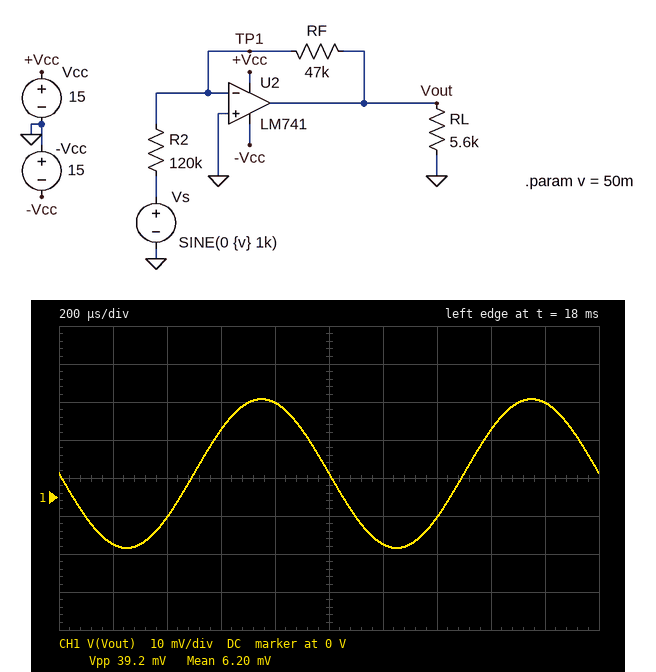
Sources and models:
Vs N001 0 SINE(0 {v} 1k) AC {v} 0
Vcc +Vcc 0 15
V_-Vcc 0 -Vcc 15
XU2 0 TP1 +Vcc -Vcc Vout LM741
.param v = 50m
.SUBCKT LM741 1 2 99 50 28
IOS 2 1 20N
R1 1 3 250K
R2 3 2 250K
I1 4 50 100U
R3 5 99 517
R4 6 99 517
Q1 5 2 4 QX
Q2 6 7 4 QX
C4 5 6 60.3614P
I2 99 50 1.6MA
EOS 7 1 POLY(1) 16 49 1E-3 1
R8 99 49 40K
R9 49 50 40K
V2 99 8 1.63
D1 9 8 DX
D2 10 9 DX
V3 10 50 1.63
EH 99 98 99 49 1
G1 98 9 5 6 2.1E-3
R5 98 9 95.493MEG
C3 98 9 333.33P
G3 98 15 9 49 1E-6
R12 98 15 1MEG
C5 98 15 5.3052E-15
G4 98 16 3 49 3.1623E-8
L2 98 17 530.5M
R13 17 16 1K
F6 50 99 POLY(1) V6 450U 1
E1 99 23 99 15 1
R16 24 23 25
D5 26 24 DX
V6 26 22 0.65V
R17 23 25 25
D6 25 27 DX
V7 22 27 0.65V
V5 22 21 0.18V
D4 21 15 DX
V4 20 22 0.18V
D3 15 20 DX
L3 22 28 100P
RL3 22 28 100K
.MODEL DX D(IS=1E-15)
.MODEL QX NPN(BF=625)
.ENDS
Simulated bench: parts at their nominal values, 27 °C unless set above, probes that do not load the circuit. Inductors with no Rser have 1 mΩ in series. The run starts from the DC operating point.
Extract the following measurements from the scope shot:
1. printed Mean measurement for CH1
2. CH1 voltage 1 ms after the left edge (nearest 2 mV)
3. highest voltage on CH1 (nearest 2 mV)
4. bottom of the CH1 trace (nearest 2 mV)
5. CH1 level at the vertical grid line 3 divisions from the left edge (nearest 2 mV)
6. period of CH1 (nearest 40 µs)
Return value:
6.20 mV
6 mV
26 mV
-14 mV
18 mV
1.00 ms
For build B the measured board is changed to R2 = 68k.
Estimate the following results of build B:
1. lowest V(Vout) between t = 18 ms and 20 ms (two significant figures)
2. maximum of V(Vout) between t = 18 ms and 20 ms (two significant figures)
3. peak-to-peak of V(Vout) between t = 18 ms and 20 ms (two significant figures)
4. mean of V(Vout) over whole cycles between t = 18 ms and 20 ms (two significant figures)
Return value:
-28 mV
41 mV
69 mV
6.5 mV
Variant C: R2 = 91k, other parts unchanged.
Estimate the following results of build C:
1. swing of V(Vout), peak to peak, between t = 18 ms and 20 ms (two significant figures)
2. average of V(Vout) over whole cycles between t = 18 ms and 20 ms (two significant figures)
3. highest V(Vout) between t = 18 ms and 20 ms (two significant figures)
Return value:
52 mV
6.3 mV
32 mV
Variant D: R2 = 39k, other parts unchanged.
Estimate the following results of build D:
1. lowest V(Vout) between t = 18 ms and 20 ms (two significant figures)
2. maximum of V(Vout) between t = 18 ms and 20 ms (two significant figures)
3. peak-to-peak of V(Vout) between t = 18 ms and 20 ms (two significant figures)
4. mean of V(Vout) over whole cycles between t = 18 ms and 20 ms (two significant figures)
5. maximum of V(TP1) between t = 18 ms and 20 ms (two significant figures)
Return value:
-53 mV
67 mV
120 mV
7.0 mV
1.1 mV
